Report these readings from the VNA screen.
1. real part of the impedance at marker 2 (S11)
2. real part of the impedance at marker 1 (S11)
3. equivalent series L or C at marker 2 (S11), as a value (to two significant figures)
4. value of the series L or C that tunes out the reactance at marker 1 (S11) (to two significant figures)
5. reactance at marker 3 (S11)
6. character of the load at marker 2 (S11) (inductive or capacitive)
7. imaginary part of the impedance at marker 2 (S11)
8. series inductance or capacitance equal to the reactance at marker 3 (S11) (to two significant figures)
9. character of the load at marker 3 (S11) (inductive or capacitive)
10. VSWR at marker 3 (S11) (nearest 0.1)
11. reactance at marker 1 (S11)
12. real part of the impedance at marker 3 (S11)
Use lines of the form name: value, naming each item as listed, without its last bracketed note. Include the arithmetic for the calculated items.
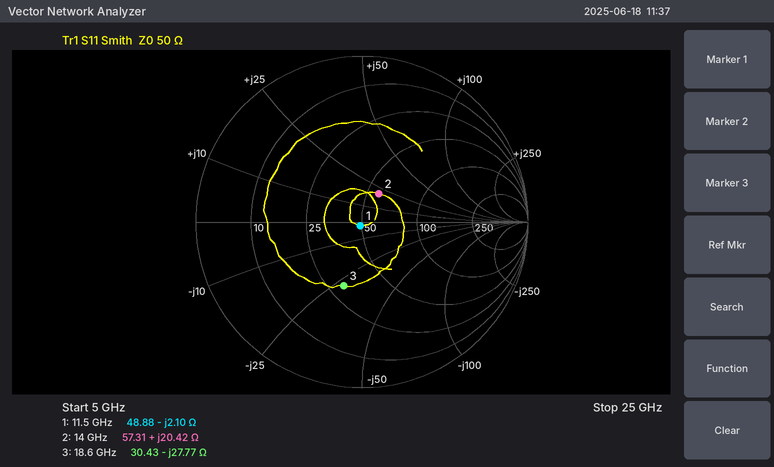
real part of the impedance at marker 2: 57.31 Ω
real part of the impedance at marker 1: 48.88 Ω
equivalent series L or C at marker 2 (S11), as a value: L = 20.42 Ω/(2π × 14 GHz) ≈ 232 pH, so 230 pH to two significant figures
value of the series L or C that tunes out the reactance at marker 1 (S11): L = 2.1 Ω/(2π × 11.5 GHz) ≈ 29 pH
reactance at marker 3: -27.77 Ω
character of the load at marker 2 (S11): inductive
imaginary part of the impedance at marker 2: +20.42 Ω
series inductance or capacitance equal to the reactance at marker 3 (S11): C = 1/(2π × 18.6 GHz × 27.77 Ω) ≈ 308 fF, so 310 fF to two significant figures
character of the load at marker 3 (S11): capacitive
VSWR at marker 3 (S11): 2.3
reactance at marker 1: -2.10 Ω
real part of the impedance at marker 3: 30.43 Ω
